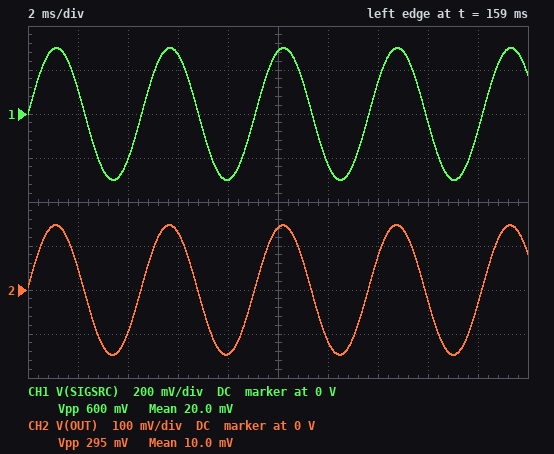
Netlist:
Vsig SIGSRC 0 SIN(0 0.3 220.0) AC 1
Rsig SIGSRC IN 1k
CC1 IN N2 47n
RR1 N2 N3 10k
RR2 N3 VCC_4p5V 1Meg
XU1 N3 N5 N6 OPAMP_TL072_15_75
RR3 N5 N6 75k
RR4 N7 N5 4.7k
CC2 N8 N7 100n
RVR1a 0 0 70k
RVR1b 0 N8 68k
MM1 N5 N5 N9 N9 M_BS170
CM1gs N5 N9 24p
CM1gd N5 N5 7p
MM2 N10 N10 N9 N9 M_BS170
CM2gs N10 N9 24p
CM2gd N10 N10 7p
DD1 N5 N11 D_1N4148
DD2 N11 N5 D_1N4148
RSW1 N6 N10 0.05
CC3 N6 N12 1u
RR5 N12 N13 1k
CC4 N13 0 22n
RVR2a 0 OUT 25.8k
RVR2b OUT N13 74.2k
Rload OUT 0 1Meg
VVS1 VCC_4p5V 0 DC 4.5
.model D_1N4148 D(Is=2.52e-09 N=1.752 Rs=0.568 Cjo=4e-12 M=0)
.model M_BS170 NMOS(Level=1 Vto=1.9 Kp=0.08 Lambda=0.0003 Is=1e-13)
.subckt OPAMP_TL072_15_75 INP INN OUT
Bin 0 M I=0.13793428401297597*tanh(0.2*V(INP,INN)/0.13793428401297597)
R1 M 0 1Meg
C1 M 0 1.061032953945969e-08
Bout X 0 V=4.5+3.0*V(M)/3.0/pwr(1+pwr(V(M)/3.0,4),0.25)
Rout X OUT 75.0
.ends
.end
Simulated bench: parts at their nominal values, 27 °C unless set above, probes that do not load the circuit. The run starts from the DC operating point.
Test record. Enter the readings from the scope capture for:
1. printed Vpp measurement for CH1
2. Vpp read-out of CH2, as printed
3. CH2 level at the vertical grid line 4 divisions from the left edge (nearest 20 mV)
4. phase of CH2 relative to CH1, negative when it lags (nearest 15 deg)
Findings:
600 mV
295 mV
-140 mV
0 deg
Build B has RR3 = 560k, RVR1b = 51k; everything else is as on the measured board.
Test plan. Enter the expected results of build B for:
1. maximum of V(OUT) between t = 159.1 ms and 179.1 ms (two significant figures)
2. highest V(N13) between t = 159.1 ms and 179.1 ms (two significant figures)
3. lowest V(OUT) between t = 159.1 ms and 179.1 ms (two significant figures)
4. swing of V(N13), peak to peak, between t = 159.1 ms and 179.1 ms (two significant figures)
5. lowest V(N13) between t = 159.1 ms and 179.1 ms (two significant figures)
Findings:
640 mV
2.5 V
-640 mV
5.1 V
-2.5 V
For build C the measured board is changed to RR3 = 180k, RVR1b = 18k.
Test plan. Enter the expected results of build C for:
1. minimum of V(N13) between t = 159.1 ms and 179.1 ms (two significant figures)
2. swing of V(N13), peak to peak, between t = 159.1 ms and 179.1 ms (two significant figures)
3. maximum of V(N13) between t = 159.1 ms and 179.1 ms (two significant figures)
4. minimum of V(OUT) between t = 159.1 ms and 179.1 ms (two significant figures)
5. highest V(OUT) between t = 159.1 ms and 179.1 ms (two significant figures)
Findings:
-2.4 V
4.9 V
2.4 V
-620 mV
620 mV
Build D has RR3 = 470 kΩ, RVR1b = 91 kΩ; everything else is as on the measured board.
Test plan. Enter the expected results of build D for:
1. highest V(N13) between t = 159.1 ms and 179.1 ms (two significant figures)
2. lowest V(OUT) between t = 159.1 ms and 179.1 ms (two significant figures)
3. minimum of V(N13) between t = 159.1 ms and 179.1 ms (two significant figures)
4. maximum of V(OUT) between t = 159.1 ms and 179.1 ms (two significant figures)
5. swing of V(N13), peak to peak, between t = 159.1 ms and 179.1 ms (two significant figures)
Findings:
1.7 V
-430 mV
-1.7 V
430 mV
3.4 V
